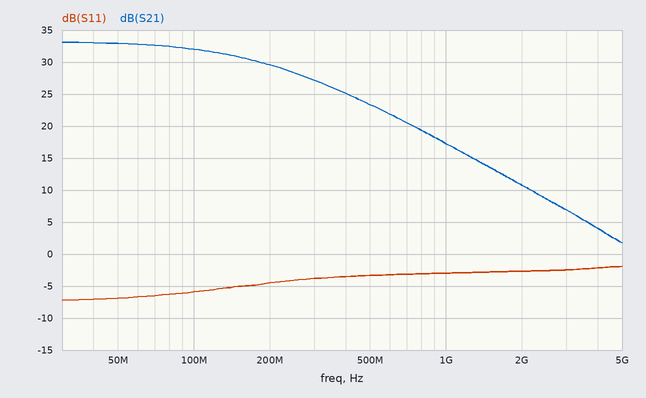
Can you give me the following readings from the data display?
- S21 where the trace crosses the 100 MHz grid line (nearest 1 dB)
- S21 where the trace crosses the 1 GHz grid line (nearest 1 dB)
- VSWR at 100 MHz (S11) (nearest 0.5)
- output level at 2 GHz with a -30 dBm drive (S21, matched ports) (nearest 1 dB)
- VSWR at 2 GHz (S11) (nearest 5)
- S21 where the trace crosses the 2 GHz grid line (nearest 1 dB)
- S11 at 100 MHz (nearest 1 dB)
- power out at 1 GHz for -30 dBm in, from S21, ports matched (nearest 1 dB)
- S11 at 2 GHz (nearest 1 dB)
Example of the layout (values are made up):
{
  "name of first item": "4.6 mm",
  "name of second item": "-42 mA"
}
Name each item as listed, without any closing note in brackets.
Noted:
{
  "S21 where the trace crosses the 100 MHz grid line": "32 dB",
  "S21 where the trace crosses the 1 GHz grid line": "17 dB",
  "VSWR at 100 MHz (S11)": "3.0",
  "output level at 2 GHz with a -30 dBm drive (S21, matched ports)": "-19 dBm",
  "VSWR at 2 GHz (S11)": "5",
  "S21 where the trace crosses the 2 GHz grid line": "11 dB",
  "S11 at 100 MHz": "-6 dB",
  "power out at 1 GHz for -30 dBm in, from S21, ports matched": "-13 dBm",
  "S11 at 2 GHz": "-3 dB"
}
